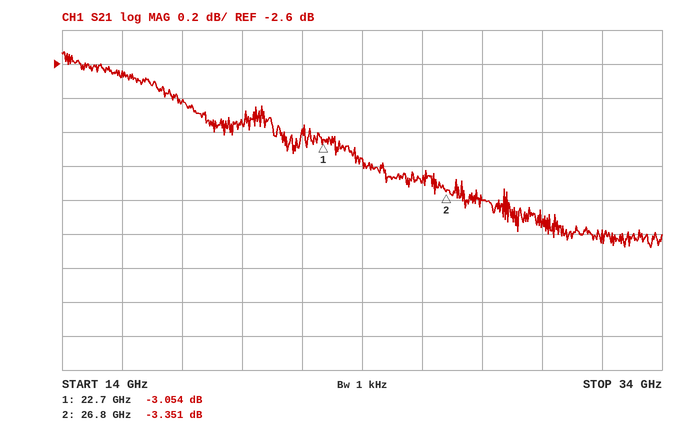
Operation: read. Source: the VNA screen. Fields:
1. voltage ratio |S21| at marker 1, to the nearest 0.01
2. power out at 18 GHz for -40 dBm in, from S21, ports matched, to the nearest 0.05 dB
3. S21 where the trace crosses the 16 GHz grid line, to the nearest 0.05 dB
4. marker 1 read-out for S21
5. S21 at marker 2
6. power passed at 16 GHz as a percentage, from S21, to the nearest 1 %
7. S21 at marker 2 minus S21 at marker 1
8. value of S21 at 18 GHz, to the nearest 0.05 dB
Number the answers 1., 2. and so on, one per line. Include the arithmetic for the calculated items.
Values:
1. 10^(-3.054/20) ≈ 0.70
2. -40 dBm + (-2.80 dB) = -42.80 dBm
3. -2.65 dB
4. -3.054 dB
5. -3.351 dB
6. 10^(-2.65/10) ≈ 54 %
7. -3.351 − (-3.054) = -0.297 dB
8. -2.80 dB
